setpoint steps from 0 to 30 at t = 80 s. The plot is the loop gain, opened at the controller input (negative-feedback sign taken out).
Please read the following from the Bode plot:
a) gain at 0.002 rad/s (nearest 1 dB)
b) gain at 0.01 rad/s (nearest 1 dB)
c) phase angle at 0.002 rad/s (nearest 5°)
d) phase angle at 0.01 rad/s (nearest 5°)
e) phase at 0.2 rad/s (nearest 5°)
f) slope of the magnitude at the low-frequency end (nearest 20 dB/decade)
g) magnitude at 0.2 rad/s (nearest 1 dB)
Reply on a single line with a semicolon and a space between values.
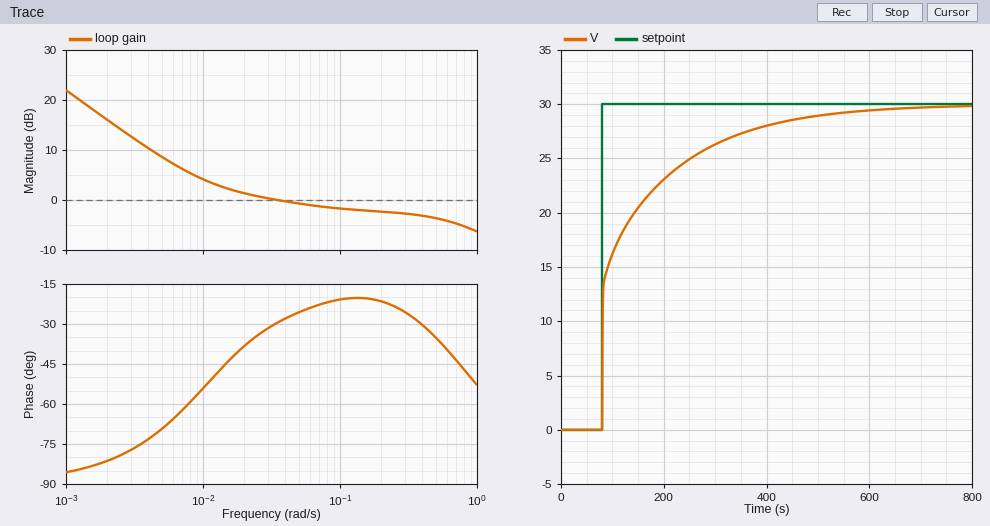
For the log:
16 dB; 4 dB; -80°; -55°; -20°; -20 dB/decade; -2 dB
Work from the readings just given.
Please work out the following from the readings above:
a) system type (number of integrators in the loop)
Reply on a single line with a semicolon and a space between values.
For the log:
1
